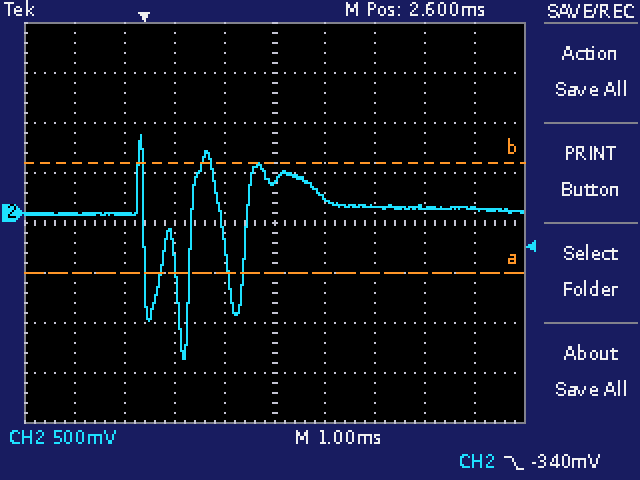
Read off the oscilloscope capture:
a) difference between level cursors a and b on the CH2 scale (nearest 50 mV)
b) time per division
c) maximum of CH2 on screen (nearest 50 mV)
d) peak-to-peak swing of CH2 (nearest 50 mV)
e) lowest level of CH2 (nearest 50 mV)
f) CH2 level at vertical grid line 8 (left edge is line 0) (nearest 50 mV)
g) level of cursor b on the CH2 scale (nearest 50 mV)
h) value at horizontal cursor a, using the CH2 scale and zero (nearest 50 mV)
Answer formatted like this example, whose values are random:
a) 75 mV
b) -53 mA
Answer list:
a) 1.10 V
b) 1 ms
c) 800 mV
d) 2.25 V
e) -1.45 V
f) 50 mV
g) 500 mV
h) -600 mV
